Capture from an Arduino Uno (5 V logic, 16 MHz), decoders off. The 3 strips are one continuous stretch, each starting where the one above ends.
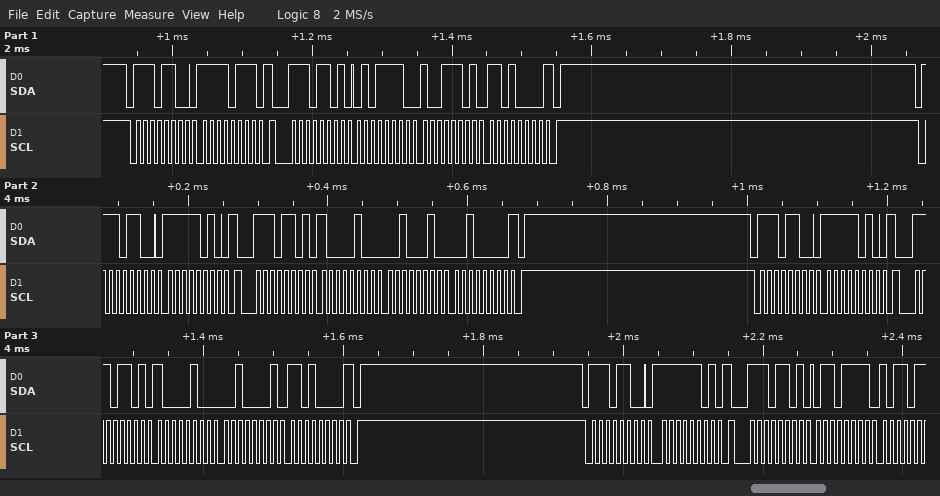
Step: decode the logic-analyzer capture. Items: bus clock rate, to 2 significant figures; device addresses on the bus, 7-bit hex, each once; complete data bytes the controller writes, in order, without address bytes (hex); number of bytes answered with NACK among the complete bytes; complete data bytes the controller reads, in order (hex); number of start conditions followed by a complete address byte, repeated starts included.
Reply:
100 kHz
0x76
F7 FA FA FD
3
5E 9D D0 84 22 20 84 21 D0 6F
8
